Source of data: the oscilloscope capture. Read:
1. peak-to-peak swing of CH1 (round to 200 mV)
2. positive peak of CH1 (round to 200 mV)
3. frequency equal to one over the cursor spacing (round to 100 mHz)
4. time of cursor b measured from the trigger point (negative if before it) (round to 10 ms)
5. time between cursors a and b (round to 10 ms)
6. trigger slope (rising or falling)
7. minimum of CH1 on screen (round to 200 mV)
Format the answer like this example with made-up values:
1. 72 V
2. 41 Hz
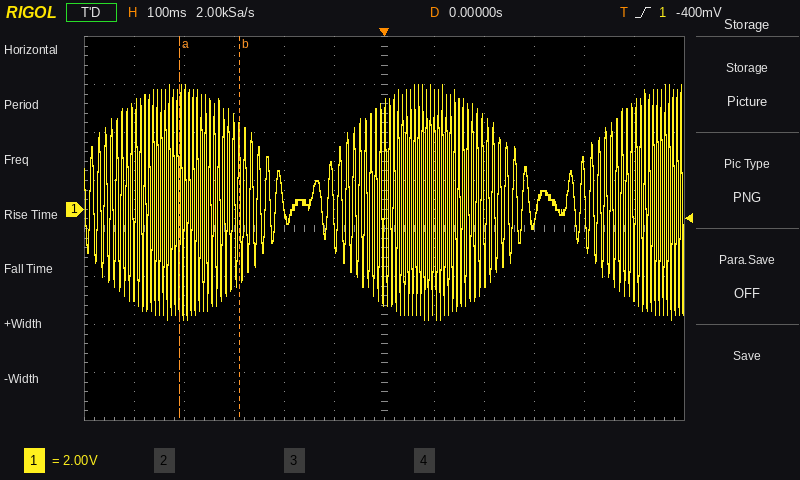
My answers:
1. 9.8 V
2. 5.2 V
3. 8.3 Hz
4. -290 ms
5. 120 ms
6. rising
7. -4.6 V
